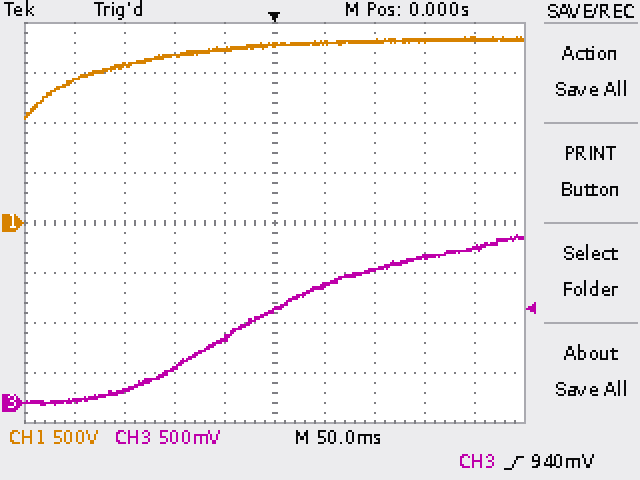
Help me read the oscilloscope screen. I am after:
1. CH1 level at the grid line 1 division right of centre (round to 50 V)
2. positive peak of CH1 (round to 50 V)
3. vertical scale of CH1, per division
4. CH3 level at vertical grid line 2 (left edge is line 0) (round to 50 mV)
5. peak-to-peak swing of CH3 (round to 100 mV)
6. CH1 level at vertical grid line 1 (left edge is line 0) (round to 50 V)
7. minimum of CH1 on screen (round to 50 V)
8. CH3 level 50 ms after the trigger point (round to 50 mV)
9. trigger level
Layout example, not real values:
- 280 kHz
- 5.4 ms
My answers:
- 1.80 kV
- 1.85 kV
- 500 V
- 100 mV
- 1.70 V
- 1.40 kV
- 1.05 kV
- 1.15 V
- 940 mV
